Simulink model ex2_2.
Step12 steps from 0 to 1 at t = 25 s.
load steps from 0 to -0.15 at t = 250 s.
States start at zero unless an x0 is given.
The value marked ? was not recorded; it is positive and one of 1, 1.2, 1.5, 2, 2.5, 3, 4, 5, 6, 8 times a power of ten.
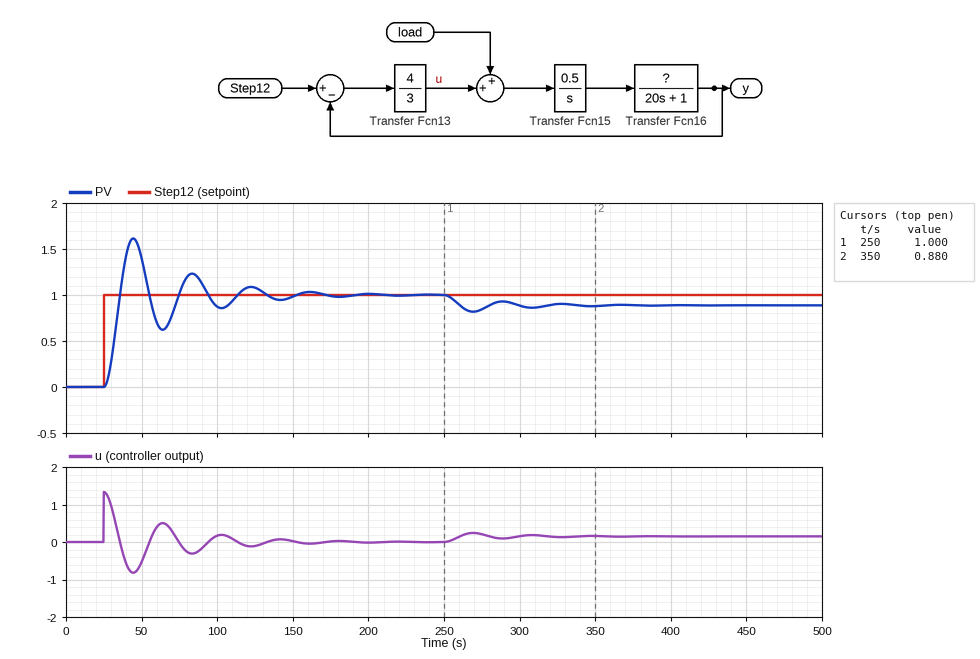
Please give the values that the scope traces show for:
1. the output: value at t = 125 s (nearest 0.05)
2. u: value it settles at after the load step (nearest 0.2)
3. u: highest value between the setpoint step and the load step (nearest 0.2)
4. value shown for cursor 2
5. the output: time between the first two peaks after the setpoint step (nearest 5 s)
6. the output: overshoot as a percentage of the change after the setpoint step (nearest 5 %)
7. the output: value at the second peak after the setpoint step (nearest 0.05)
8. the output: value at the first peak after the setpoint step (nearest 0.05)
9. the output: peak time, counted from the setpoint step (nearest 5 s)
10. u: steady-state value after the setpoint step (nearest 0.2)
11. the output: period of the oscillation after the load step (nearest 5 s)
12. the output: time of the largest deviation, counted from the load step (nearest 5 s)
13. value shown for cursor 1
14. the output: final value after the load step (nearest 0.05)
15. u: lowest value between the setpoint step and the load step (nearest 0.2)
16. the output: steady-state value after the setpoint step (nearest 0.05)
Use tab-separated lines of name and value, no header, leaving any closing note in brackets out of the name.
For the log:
the output: value at t = 125 s	1.10
u: value it settles at after the load step	0.2
u: highest value between the setpoint step and the load step	1.4
value shown for cursor 2	0.880
the output: time between the first two peaks after the setpoint step	40 s
the output: overshoot as a percentage of the change after the setpoint step	60 %
the output: value at the second peak after the setpoint step	1.25
the output: value at the first peak after the setpoint step	1.60
the output: peak time, counted from the setpoint step	20 s
u: steady-state value after the setpoint step	0.0
the output: period of the oscillation after the load step	40 s
the output: time of the largest deviation, counted from the load step	20 s
value shown for cursor 1	1.000
the output: final value after the load step	0.90
u: lowest value between the setpoint step and the load step	-0.8
the output: steady-state value after the setpoint step	1.00
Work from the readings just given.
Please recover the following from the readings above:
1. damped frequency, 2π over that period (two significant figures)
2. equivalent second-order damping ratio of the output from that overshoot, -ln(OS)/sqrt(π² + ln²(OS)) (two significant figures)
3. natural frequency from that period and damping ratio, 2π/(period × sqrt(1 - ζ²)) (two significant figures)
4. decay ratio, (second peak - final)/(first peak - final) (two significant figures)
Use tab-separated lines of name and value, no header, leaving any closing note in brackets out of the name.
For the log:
damped frequency, 2π over that period	0.16 rad/s
equivalent second-order damping ratio of the output from that overshoot, -ln(OS)/sqrt(π² + ln²(OS))	0.16
natural frequency from that period and damping ratio, 2π/(period × sqrt(1 - ζ²))	0.16 rad/s
decay ratio, (second peak - final)/(first peak - final)	0.42
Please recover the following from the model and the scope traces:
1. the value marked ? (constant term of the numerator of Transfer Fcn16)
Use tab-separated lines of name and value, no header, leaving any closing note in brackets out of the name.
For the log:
the value marked ?	0.8
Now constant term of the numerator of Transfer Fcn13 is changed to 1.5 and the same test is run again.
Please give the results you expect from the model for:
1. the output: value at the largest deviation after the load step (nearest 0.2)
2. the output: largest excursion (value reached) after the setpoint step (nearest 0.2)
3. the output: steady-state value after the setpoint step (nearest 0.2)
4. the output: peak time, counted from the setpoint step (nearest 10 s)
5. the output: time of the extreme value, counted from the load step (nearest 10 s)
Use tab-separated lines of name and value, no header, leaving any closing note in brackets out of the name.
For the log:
the output: value at the largest deviation after the load step	0.6
the output: largest excursion (value reached) after the setpoint step	1.4
the output: steady-state value after the setpoint step	1.0
the output: peak time, counted from the setpoint step	30 s
the output: time of the extreme value, counted from the load step	30 s
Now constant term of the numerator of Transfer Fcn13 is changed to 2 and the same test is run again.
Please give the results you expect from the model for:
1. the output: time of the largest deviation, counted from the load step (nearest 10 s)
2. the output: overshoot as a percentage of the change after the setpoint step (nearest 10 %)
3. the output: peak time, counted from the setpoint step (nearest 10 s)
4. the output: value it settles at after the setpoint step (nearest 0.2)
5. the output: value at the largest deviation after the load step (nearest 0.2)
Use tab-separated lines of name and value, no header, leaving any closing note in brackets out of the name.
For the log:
the output: time of the largest deviation, counted from the load step	30 s
the output: overshoot as a percentage of the change after the setpoint step	50 %
the output: peak time, counted from the setpoint step	30 s
the output: value it settles at after the setpoint step	1.0
the output: value at the largest deviation after the load step	0.6
